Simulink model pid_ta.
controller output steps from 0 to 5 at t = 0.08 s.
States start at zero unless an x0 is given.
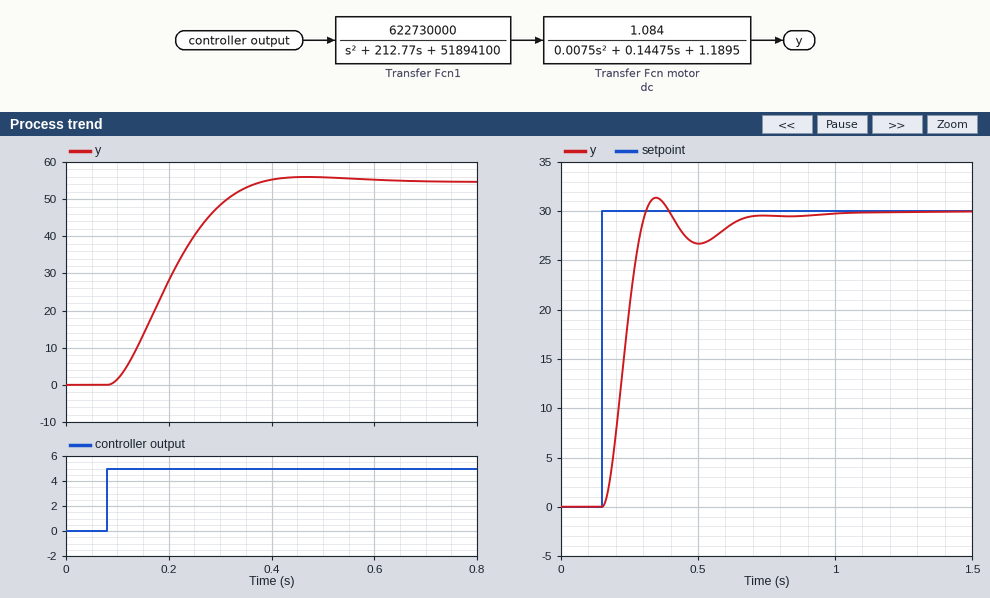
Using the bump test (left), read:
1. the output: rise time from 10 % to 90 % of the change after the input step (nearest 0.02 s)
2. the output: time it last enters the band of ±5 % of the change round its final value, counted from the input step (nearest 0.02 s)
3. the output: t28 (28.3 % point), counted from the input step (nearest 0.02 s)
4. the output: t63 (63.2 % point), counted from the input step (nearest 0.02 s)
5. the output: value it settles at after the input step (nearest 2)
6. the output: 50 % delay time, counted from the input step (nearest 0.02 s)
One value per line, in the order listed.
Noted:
0.18 s
0.26 s
0.08 s
0.14 s
54
0.12 s
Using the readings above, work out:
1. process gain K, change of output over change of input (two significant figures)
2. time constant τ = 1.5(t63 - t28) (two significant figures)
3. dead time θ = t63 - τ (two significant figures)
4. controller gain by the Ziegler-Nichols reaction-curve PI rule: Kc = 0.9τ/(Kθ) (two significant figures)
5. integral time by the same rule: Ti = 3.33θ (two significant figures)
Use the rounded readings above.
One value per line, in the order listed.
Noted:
11
0.090 s
0.050 s
0.15
0.17 s
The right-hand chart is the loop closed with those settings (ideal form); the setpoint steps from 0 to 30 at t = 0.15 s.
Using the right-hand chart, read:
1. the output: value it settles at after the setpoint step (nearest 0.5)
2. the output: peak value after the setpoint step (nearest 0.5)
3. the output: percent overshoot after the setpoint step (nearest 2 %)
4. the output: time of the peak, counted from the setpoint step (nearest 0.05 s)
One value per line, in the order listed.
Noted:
30.0
31.5
4 %
0.20 s
